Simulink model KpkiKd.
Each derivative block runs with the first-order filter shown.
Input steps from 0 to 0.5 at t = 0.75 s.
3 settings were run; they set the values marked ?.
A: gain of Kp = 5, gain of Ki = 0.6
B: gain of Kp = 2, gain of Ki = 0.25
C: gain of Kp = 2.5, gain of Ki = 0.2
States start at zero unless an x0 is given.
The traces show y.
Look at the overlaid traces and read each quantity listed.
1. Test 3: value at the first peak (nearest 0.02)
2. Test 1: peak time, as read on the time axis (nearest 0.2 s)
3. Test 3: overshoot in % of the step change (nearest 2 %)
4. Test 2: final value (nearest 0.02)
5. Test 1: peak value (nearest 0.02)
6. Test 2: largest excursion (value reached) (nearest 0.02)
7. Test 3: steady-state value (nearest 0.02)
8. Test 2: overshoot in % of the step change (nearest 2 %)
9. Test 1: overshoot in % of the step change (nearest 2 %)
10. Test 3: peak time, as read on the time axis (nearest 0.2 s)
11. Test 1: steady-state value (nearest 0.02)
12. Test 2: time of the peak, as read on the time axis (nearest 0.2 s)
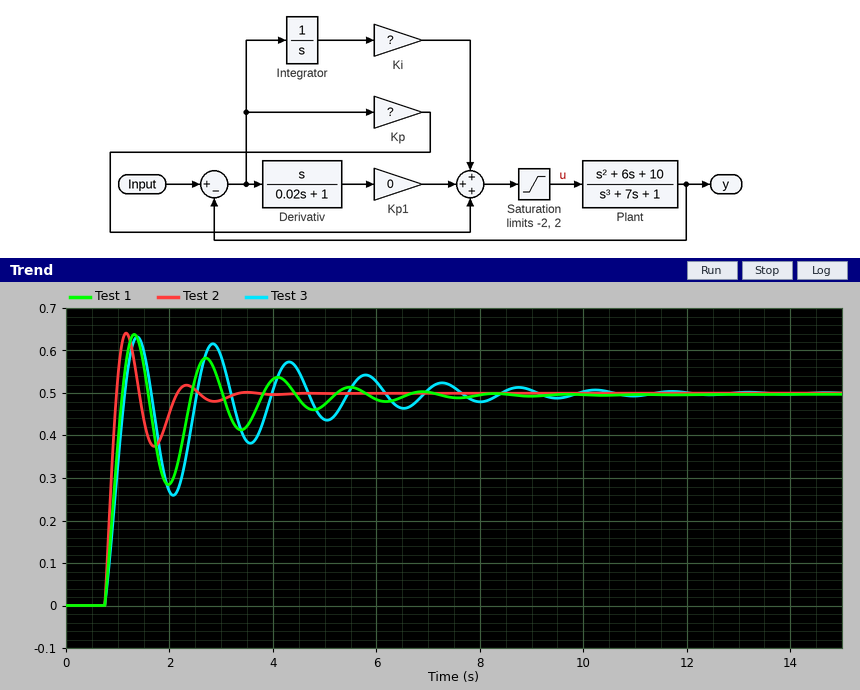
0.64
1.4 s
26 %
0.50
0.64
0.64
0.50
28 %
28 %
1.4 s
0.50
1.2 s
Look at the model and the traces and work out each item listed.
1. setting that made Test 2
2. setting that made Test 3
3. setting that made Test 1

A
B
C
